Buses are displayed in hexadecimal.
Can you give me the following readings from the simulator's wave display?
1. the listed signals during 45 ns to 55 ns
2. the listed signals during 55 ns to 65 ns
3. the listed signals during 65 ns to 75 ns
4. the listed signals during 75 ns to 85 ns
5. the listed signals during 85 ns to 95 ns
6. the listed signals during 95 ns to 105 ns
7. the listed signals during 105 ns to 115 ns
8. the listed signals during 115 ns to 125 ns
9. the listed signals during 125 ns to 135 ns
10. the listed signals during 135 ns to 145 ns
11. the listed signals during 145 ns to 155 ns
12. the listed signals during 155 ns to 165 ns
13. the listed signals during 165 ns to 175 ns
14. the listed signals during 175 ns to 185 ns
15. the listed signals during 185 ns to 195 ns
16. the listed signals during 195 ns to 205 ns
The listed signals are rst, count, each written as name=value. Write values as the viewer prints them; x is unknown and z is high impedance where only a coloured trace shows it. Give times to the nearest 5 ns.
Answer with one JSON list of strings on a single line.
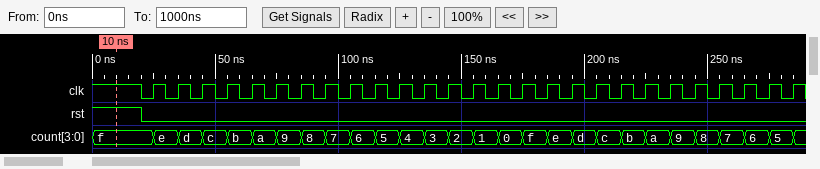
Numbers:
["rst=0, count=c", "rst=0, count=b", "rst=0, count=a", "rst=0, count=9", "rst=0, count=8", "rst=0, count=7", "rst=0, count=6", "rst=0, count=5", "rst=0, count=4", "rst=0, count=3", "rst=0, count=2", "rst=0, count=1", "rst=0, count=0", "rst=0, count=f", "rst=0, count=e", "rst=0, count=d"]
